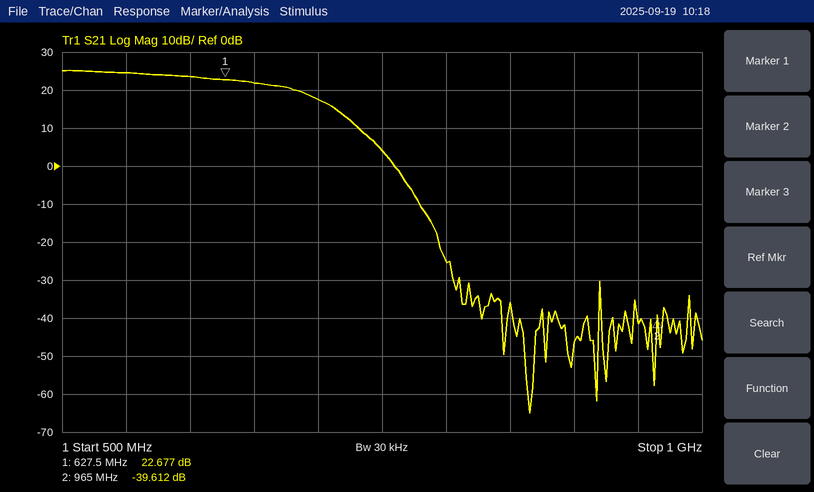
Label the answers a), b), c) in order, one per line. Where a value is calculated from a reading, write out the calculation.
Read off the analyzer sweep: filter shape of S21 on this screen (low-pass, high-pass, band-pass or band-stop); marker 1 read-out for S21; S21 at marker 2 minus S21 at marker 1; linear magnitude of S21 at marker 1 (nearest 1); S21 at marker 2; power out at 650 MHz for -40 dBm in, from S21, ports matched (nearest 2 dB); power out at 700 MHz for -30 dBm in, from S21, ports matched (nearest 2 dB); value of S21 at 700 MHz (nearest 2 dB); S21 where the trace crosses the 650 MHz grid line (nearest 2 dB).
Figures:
a) low-pass
b) 22.677 dB
c) -39.612 − (22.677) = -62.289 dB
d) 10^(22.677/20) ≈ 14
e) -39.612 dB
f) -40 dBm + (22 dB) = -18 dBm
g) -30 dBm + (18 dB) = -12 dBm
h) 18 dB
i) 22 dB
